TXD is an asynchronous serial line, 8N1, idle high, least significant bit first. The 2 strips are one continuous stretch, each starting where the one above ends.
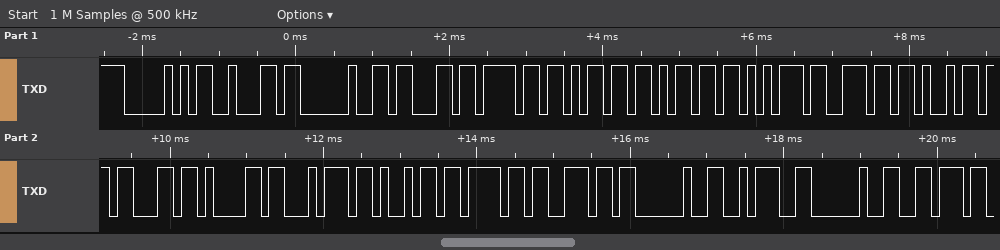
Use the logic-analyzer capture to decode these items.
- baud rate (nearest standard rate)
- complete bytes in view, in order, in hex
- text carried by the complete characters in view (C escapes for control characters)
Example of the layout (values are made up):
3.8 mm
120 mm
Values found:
9600 baud
50 62 20 63 6F 6D 6D 75 6E 69 63 61 74 69 6F 6E 20 3A 20 76
"Pb communication : v"
